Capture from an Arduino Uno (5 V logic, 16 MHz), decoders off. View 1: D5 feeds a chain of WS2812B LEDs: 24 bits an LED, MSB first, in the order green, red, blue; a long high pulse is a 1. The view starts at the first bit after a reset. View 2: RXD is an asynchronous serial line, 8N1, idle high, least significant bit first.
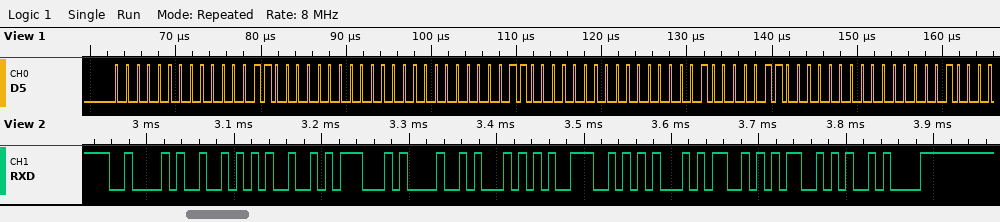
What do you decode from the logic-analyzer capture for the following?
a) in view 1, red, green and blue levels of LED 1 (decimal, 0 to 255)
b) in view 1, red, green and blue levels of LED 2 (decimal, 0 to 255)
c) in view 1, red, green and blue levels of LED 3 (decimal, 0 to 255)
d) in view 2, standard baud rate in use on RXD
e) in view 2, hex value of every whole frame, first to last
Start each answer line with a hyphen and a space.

- 6, 0, 0
- 6, 0, 0
- 6, 1, 0
- 115200 baud
- 0x42 0x52 0x49 0x47 0x48 0x54 0x4E 0x45 0x53 0x53 0x0A
